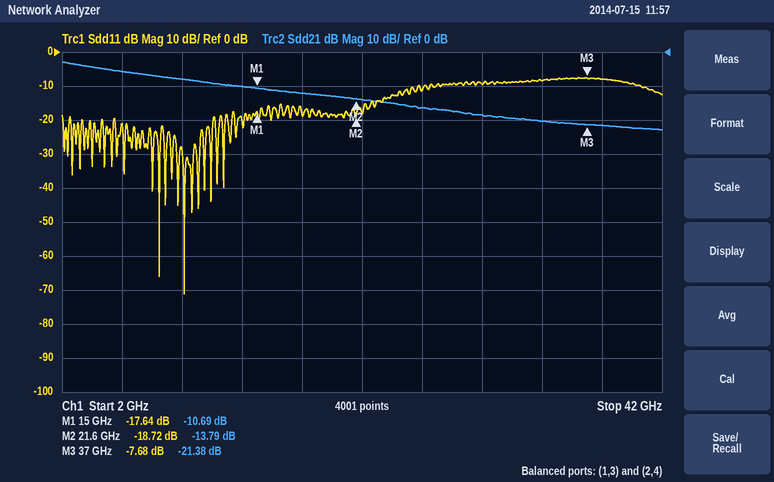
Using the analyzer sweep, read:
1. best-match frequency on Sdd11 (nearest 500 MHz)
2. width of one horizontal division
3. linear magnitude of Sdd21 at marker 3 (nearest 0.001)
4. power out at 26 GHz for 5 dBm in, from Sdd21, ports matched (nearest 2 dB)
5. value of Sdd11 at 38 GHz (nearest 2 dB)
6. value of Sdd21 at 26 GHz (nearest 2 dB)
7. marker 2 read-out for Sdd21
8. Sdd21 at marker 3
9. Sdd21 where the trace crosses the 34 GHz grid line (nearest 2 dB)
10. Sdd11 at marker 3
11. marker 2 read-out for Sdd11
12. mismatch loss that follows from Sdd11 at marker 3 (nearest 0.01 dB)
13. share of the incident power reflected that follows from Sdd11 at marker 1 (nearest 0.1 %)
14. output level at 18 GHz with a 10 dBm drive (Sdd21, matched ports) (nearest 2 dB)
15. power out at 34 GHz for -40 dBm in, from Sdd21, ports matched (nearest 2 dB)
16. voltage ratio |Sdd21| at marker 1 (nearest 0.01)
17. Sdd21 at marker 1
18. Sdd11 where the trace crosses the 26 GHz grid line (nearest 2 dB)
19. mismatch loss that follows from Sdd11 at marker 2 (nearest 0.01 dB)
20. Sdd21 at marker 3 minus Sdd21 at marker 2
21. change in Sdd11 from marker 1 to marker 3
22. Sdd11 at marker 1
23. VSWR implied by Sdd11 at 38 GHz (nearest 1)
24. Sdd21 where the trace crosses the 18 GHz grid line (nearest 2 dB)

10.0 GHz
4 GHz
0.085
-12 dBm
-8 dB
-16 dB
-13.79 dB
-21.38 dB
-20 dB
-7.68 dB
-18.72 dB
0.81 dB
1.7 %
-2 dBm
-60 dBm
0.29
-10.69 dB
-12 dB
0.06 dB
-7.59 dB
9.96 dB
-17.64 dB
2
-12 dB
